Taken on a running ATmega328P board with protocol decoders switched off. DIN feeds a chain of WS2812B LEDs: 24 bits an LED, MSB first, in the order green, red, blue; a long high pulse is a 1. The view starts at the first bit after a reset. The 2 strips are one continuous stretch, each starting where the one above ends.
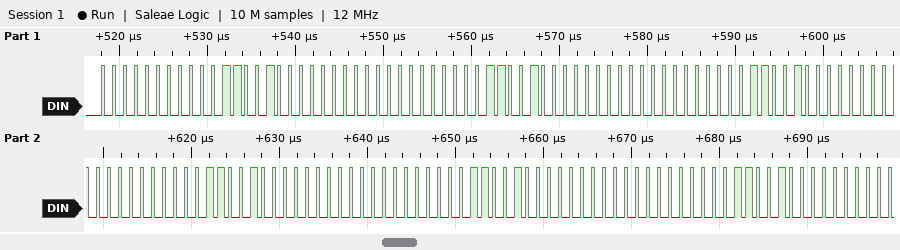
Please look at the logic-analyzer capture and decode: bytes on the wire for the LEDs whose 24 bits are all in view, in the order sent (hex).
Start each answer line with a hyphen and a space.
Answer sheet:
- 00 19 00 00 19 00 00 19 00 00 19 00 00 19 00 00 19 00
